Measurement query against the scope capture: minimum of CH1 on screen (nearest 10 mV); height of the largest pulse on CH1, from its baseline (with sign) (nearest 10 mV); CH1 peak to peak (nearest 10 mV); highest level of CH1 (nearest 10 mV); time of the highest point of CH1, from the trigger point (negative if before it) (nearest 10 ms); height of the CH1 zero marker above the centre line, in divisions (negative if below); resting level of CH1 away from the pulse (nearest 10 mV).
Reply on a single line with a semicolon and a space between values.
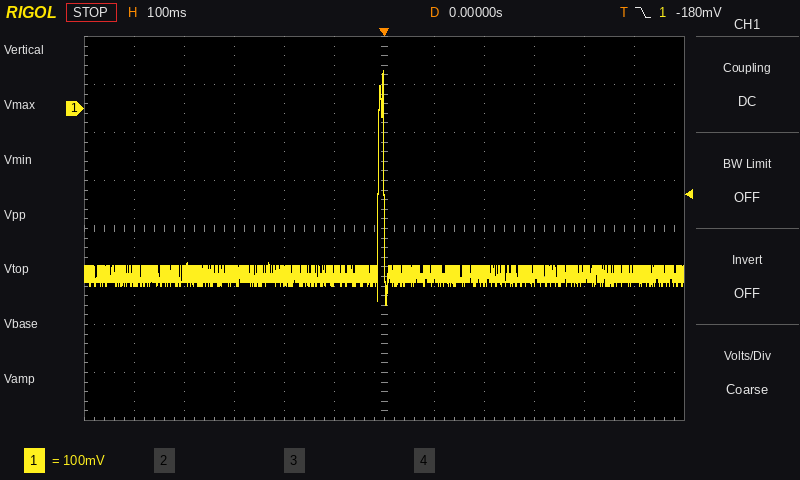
-410 mV; +420 mV; 490 mV; 80 mV; 0 ms; +2.5 div; -340 mV
